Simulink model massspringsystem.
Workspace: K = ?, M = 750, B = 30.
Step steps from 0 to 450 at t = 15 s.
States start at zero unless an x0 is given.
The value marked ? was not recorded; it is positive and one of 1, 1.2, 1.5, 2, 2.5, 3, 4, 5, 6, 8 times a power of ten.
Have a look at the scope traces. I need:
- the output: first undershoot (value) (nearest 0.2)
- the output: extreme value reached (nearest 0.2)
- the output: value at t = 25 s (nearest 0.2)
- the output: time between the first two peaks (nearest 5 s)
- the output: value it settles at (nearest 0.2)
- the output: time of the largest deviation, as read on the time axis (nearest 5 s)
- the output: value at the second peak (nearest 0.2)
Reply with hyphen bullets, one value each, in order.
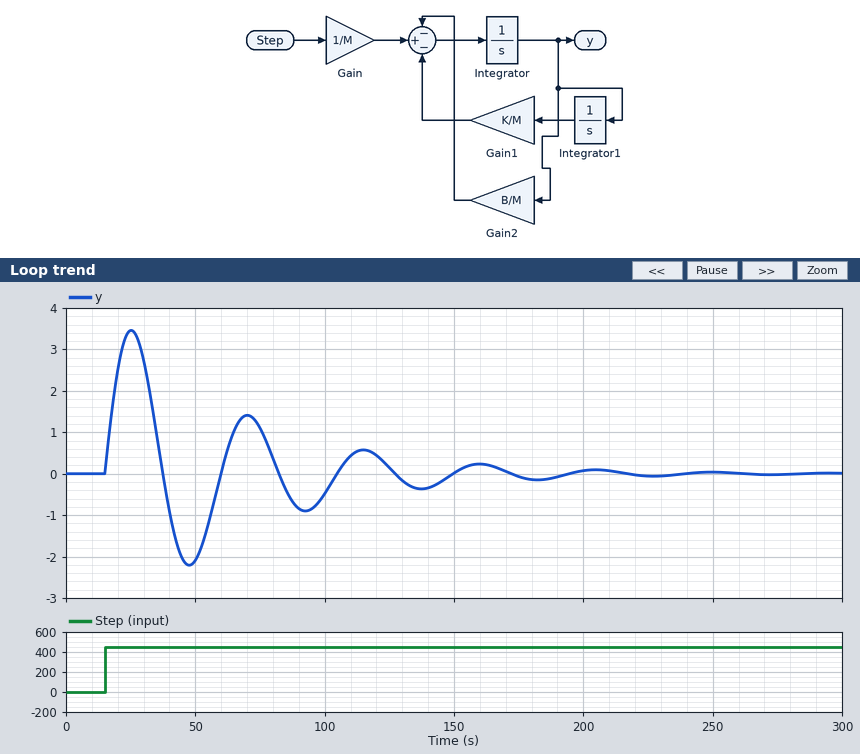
- -2.2
- 3.4
- 3.4
- 45 s
- 0.0
- 25 s
- 1.4
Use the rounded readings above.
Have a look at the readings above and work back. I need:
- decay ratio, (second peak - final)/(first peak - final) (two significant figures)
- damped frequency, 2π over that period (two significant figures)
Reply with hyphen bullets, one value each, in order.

- 0.41
- 0.14 rad/s
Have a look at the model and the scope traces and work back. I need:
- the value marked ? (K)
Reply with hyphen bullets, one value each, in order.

- 15
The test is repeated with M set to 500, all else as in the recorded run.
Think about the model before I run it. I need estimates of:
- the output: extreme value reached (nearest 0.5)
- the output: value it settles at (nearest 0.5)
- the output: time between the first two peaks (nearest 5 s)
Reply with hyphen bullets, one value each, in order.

- 4.0
- 0.0
- 35 s
